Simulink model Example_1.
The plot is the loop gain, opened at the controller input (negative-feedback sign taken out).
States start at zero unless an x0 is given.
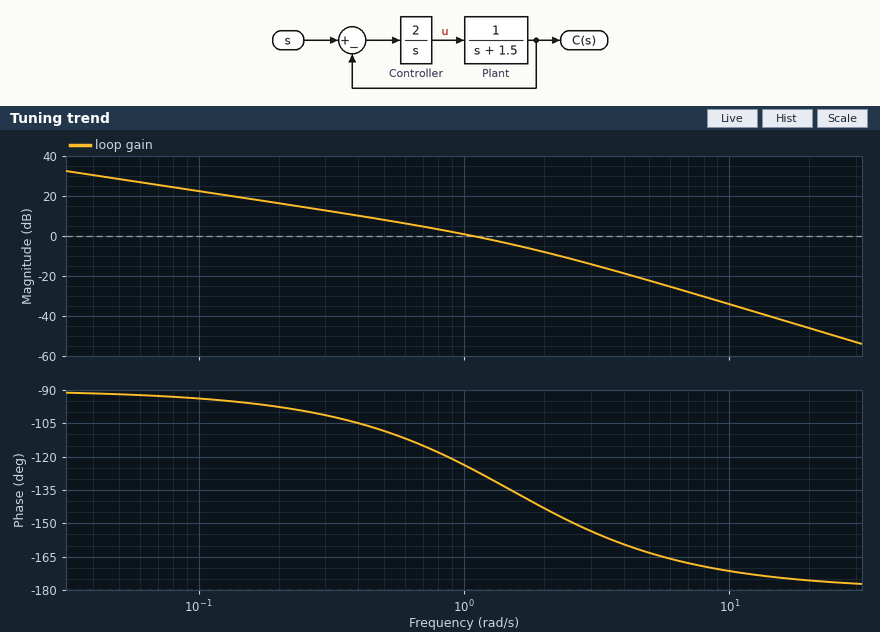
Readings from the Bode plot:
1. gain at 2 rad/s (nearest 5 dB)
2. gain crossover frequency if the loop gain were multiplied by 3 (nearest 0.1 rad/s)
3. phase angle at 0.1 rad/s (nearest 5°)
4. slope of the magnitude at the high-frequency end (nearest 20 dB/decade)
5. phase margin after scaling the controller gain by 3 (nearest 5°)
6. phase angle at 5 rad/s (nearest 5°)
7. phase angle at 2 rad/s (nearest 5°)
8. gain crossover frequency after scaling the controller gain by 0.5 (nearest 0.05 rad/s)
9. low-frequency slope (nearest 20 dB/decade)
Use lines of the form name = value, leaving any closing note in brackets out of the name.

gain at 2 rad/s = -10 dB
gain crossover frequency if the loop gain were multiplied by 3 = 2.2 rad/s
phase angle at 0.1 rad/s = -95°
slope of the magnitude at the high-frequency end = -40 dB/decade
phase margin after scaling the controller gain by 3 = 35°
phase angle at 5 rad/s = -165°
phase angle at 2 rad/s = -145°
gain crossover frequency after scaling the controller gain by 0.5 = 0.60 rad/s
low-frequency slope = -20 dB/decade
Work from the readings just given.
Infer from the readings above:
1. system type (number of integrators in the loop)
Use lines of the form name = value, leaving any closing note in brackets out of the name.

system type = 1
